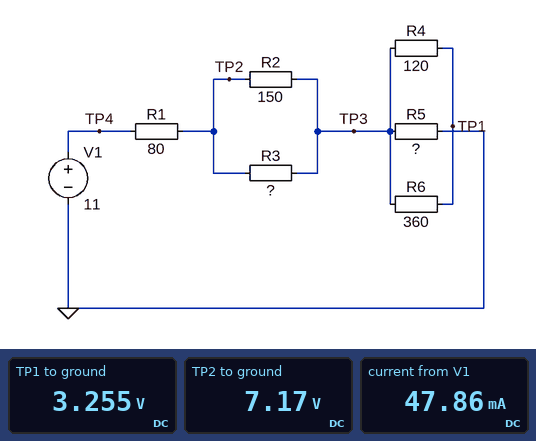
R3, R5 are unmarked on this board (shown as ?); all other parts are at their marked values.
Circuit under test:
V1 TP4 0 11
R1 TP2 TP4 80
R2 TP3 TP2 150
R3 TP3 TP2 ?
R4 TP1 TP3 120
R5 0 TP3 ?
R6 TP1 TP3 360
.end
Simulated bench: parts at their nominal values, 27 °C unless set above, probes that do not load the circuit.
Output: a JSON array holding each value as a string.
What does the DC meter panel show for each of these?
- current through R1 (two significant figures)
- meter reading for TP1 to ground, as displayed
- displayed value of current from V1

["48 mA", "3.255 V", "47.86 mA"]
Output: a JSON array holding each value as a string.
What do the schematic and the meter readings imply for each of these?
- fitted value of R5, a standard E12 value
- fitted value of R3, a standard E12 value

["68 Ω", "180 Ω"]
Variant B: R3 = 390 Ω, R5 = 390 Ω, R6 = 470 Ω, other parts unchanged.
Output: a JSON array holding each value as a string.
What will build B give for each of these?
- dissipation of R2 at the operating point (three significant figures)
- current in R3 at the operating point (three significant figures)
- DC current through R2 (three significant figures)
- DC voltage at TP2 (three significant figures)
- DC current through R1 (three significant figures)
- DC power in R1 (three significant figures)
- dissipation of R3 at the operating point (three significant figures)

["28.3 mW", "5.28 mA", "13.7 mA", "9.48 V", "19.0 mA", "28.9 mW", "10.9 mW"]
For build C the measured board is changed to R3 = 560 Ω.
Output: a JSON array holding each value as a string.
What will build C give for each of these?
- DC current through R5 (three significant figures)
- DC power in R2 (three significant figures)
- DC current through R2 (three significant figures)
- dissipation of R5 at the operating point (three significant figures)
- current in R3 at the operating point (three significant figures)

["41.3 mA", "159 mW", "32.6 mA", "116 mW", "8.73 mA"]
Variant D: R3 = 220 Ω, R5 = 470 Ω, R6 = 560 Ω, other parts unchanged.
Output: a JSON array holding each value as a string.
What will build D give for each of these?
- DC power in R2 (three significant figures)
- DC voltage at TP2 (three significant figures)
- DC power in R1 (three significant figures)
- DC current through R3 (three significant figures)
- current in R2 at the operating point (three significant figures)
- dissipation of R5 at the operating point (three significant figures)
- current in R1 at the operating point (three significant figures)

["15.7 mW", "9.62 V", "23.7 mW", "6.98 mA", "10.2 mA", "139 mW", "17.2 mA"]
